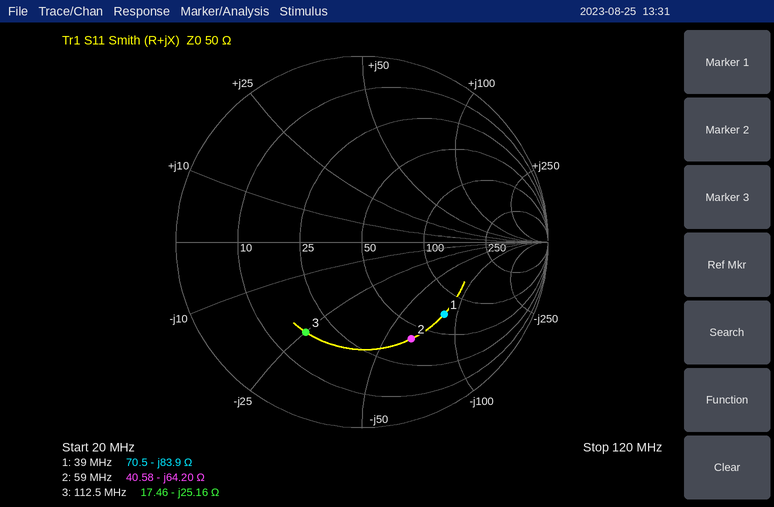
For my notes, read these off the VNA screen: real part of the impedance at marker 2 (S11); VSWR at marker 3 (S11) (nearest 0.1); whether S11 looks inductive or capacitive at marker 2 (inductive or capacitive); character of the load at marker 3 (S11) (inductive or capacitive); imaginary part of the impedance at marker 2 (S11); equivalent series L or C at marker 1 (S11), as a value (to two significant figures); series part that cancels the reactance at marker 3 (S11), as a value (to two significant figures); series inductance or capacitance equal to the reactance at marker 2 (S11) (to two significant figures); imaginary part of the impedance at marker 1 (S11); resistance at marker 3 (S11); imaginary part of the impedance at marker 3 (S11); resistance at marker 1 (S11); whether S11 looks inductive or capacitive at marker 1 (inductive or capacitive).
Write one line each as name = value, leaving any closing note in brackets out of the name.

real part of the impedance at marker 2 = 40.58 Ω
VSWR at marker 3 (S11) = 3.7
whether S11 looks inductive or capacitive at marker 2 = capacitive
character of the load at marker 3 (S11) = capacitive
imaginary part of the impedance at marker 2 = -64.20 Ω
equivalent series L or C at marker 1 (S11), as a value = 49 pF
series part that cancels the reactance at marker 3 (S11), as a value = 36 nH
series inductance or capacitance equal to the reactance at marker 2 (S11) = 42 pF
imaginary part of the impedance at marker 1 = -83.9 Ω
resistance at marker 3 = 17.46 Ω
imaginary part of the impedance at marker 3 = -25.16 Ω
resistance at marker 1 = 70.5 Ω
whether S11 looks inductive or capacitive at marker 1 = capacitive
